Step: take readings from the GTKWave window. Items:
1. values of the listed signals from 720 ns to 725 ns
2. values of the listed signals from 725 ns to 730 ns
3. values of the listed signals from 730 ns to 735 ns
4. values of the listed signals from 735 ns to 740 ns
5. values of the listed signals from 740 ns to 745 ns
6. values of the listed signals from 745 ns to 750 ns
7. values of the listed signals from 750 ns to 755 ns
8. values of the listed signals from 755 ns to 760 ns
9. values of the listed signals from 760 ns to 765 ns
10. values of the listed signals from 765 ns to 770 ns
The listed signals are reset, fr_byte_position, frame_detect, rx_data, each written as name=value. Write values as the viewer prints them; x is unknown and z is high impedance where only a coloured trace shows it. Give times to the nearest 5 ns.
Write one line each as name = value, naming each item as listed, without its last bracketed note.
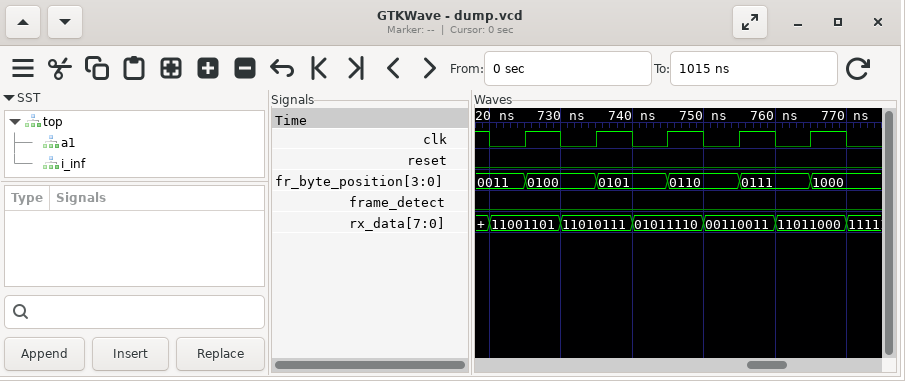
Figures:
values of the listed signals from 720 ns to 725 ns = reset=0, fr_byte_position=0011, frame_detect=0, rx_data=11001101
values of the listed signals from 725 ns to 730 ns = reset=0, fr_byte_position=0100, frame_detect=0, rx_data=11001101
values of the listed signals from 730 ns to 735 ns = reset=0, fr_byte_position=0100, frame_detect=0, rx_data=11010111
values of the listed signals from 735 ns to 740 ns = reset=0, fr_byte_position=0101, frame_detect=0, rx_data=11010111
values of the listed signals from 740 ns to 745 ns = reset=0, fr_byte_position=0101, frame_detect=0, rx_data=01011110
values of the listed signals from 745 ns to 750 ns = reset=0, fr_byte_position=0110, frame_detect=0, rx_data=01011110
values of the listed signals from 750 ns to 755 ns = reset=0, fr_byte_position=0110, frame_detect=0, rx_data=00110011
values of the listed signals from 755 ns to 760 ns = reset=0, fr_byte_position=0111, frame_detect=0, rx_data=00110011
values of the listed signals from 760 ns to 765 ns = reset=0, fr_byte_position=0111, frame_detect=0, rx_data=11011000
values of the listed signals from 765 ns to 770 ns = reset=0, fr_byte_position=1000, frame_detect=0, rx_data=11011000
